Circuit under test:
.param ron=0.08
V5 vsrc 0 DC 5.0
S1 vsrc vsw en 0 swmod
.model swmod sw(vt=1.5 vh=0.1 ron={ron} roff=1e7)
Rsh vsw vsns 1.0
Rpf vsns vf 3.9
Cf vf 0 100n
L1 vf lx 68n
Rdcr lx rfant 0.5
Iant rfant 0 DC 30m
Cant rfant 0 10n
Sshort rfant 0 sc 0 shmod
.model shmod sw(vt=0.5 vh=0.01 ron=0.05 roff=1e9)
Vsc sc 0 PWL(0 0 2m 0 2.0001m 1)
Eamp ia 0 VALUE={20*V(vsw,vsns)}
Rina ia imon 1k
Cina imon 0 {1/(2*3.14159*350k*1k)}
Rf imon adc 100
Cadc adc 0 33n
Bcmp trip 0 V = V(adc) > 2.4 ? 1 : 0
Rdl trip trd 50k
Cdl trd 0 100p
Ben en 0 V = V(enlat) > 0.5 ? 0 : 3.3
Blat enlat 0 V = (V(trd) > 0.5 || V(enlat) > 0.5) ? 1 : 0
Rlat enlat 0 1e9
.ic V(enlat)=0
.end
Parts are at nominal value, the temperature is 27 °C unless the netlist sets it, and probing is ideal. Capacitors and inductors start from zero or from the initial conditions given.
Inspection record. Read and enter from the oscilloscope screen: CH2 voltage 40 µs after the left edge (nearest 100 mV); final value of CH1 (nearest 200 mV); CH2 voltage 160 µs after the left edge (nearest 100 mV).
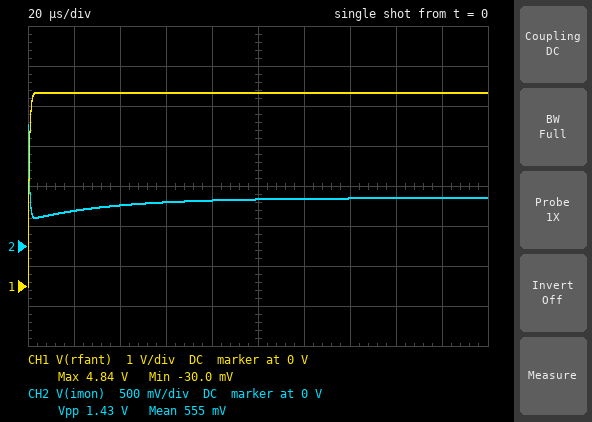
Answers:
500 mV
4.8 V
600 mV
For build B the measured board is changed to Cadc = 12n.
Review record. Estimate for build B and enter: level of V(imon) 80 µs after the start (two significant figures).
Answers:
600 mV
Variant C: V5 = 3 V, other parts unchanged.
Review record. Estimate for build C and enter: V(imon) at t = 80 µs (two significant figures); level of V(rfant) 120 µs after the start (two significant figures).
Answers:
560 mV
2.8 V
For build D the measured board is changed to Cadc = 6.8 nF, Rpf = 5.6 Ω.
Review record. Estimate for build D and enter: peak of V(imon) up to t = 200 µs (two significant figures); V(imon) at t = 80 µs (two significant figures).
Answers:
1.3 V
600 mV
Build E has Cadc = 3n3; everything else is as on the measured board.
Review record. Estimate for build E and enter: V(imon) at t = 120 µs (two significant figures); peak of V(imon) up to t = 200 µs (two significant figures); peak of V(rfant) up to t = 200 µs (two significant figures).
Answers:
600 mV
2.2 V
4.8 V
